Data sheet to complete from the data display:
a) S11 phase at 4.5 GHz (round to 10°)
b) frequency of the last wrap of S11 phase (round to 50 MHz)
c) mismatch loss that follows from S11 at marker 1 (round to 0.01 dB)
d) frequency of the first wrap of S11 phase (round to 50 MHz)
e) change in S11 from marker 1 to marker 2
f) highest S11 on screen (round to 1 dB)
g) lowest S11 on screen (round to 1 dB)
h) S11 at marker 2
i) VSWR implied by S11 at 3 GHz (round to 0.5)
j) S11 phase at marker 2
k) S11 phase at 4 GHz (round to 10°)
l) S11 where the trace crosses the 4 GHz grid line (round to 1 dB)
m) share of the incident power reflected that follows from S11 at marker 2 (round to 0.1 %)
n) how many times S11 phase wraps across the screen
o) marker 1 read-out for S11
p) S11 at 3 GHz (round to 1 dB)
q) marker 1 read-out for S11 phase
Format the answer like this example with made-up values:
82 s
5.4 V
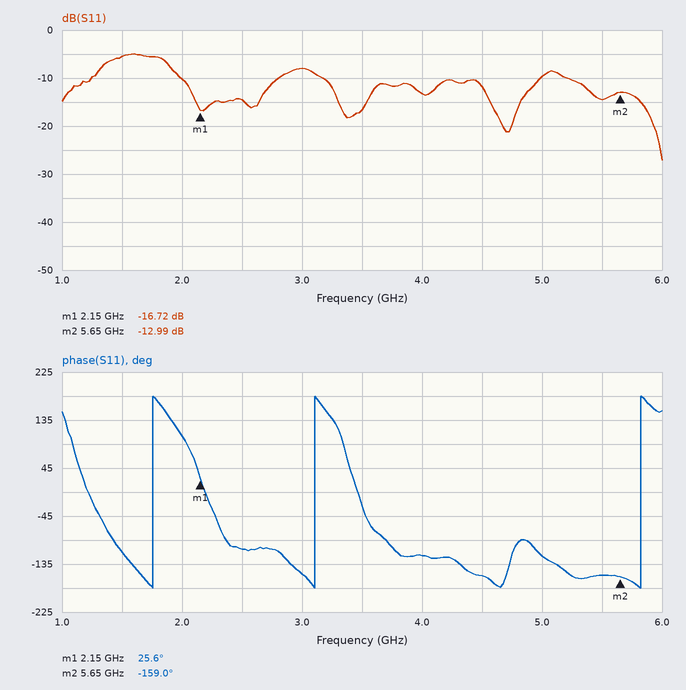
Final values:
-160°
5.80 GHz
0.09 dB
1.75 GHz
3.73 dB
-5 dB
-27 dB
-12.99 dB
2.5
-159.0°
-120°
-13 dB
5.0 %
3
-16.72 dB
-8 dB
25.6°
